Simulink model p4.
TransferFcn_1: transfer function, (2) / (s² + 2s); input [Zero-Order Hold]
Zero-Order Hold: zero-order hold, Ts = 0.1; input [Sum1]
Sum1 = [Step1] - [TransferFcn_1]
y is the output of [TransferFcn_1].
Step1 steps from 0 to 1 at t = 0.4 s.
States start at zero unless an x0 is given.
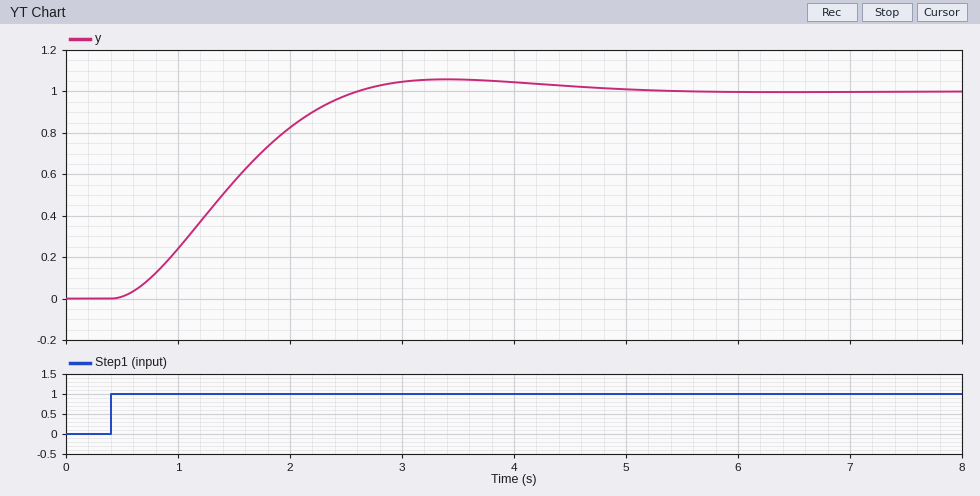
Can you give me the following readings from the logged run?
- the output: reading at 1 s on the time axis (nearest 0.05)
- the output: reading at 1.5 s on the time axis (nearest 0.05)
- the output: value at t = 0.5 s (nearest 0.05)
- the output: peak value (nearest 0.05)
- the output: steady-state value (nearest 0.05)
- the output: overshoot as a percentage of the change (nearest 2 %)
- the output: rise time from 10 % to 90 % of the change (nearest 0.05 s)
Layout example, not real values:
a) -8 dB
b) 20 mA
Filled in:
a) 0.25
b) 0.55
c) 0.00
d) 1.05
e) 1.00
f) 6 %
g) 1.45 s
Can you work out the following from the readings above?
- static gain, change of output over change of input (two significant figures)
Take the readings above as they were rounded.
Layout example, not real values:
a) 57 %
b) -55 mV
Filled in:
a) 1.0
